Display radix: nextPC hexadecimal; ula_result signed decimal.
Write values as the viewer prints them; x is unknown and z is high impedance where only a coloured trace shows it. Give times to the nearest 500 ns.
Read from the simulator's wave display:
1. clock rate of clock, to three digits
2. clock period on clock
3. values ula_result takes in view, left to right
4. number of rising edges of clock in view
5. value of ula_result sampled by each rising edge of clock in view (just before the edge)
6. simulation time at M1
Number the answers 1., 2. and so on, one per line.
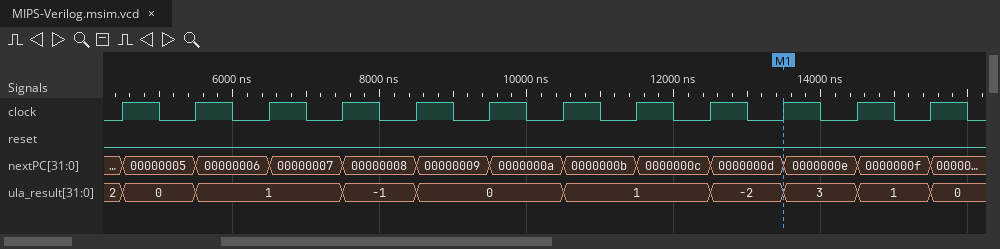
1. 1.00 MHz
2. 1000 ns
3. 2, 0, 1, -1, 0, 1, -2, 3, 1, 0
4. 12
5. 2, 0, 1, 1, -1, 0, 0, 1, 1, -2, 3, 1
6. 13500 ns
